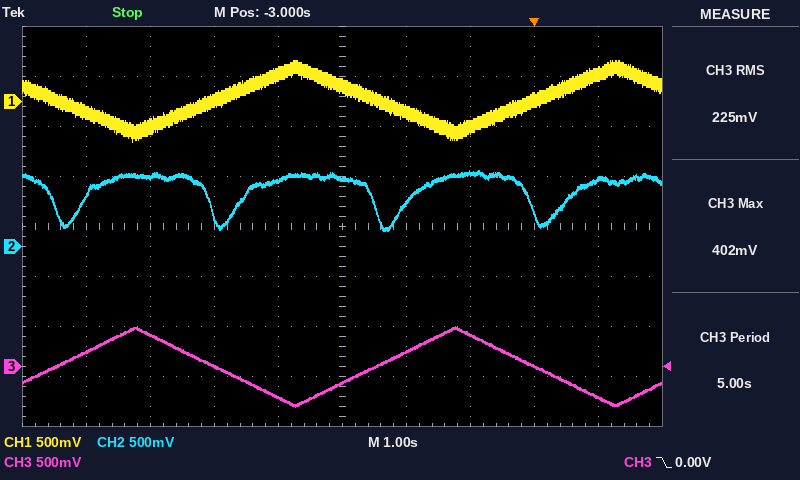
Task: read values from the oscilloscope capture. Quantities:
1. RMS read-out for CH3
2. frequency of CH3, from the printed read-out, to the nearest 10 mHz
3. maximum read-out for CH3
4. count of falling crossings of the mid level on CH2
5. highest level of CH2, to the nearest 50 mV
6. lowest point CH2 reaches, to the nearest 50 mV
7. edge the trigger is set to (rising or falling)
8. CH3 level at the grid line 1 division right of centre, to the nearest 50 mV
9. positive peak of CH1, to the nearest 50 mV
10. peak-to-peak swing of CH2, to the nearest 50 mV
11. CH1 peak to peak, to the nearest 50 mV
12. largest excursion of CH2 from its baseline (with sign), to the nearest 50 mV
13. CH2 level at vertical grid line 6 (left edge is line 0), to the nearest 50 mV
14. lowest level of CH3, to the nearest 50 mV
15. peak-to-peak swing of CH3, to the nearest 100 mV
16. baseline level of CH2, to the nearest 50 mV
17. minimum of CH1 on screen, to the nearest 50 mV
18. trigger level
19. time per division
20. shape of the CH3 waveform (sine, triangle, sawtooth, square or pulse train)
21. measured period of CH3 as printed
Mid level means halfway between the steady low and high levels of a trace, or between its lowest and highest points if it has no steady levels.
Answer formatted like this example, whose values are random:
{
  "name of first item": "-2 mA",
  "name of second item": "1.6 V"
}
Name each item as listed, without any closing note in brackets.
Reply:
{
  "RMS read-out for CH3": "225 mV",
  "frequency of CH3, from the printed read-out, to the nearest 10 mHz": "200 mHz",
  "maximum read-out for CH3": "402 mV",
  "count of falling crossings of the mid level on CH2": "4",
  "highest level of CH2, to the nearest 50 mV": "750 mV",
  "lowest point CH2 reaches, to the nearest 50 mV": "150 mV",
  "edge the trigger is set to": "falling",
  "CH3 level at the grid line 1 division right of centre, to the nearest 50 mV": "150 mV",
  "positive peak of CH1, to the nearest 50 mV": "400 mV",
  "peak-to-peak swing of CH2, to the nearest 50 mV": "600 mV",
  "CH1 peak to peak, to the nearest 50 mV": "800 mV",
  "largest excursion of CH2 from its baseline (with sign), to the nearest 50 mV": "-500 mV",
  "CH2 level at vertical grid line 6 (left edge is line 0), to the nearest 50 mV": "450 mV",
  "lowest level of CH3, to the nearest 50 mV": "-400 mV",
  "peak-to-peak swing of CH3, to the nearest 100 mV": "800 mV",
  "baseline level of CH2, to the nearest 50 mV": "650 mV",
  "minimum of CH1 on screen, to the nearest 50 mV": "-400 mV",
  "trigger level": "0.00 V",
  "time per division": "1 s",
  "shape of the CH3 waveform": "triangle",
  "measured period of CH3 as printed": "5.00 s"
}
